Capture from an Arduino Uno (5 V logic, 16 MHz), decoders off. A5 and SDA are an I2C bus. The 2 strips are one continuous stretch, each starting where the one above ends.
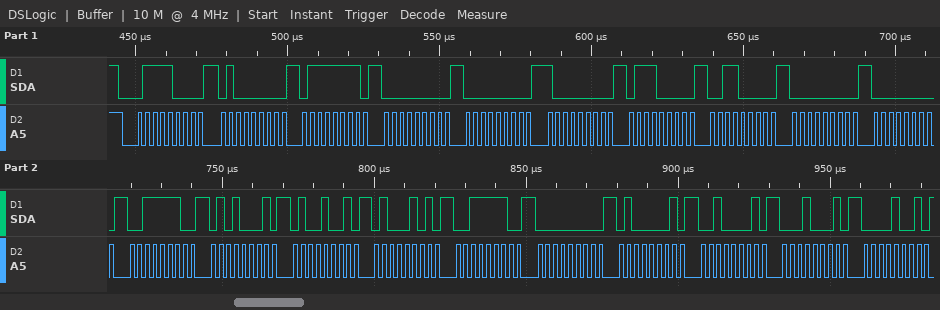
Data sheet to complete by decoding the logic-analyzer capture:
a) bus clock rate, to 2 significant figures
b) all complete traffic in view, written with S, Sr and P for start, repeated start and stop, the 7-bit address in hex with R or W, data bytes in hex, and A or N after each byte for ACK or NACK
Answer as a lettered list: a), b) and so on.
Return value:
a) 400 kHz
b) S 3CW A 40 A 7F A 00 A 00 A 80 A 70 A 30 A 00 A 00 A 3E A 51 A 49 A 45 A 3E A 00 A 41 A 21 A 11 A 09 A
